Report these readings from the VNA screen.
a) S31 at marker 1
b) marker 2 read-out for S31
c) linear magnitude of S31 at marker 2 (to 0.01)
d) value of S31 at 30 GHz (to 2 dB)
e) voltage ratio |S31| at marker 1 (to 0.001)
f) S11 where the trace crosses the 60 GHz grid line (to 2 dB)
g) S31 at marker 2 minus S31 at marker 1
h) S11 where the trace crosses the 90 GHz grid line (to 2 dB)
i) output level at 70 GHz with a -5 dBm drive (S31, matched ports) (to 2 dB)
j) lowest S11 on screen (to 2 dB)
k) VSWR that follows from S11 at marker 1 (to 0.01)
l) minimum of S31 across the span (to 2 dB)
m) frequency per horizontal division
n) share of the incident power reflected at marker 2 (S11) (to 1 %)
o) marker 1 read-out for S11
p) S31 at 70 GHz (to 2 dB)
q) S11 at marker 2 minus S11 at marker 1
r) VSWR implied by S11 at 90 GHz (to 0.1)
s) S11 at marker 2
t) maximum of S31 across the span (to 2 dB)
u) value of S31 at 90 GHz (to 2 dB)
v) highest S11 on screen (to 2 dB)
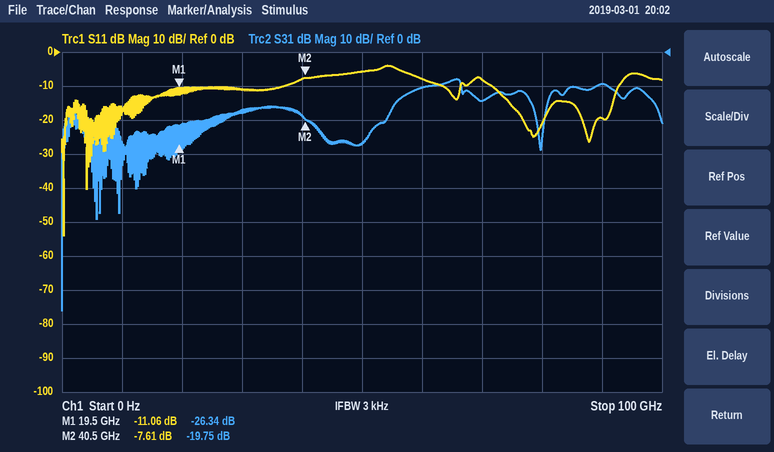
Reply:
-26.34 dB
-19.75 dB
0.10
-18 dB
0.048
-8 dB
6.59 dB
-20 dB
-20 dBm
-54 dB
1.78
-76 dB
10 GHz
17 %
-11.06 dB
-14 dB
3.45 dB
1.2
-7.61 dB
-8 dB
-10 dB
-4 dB
